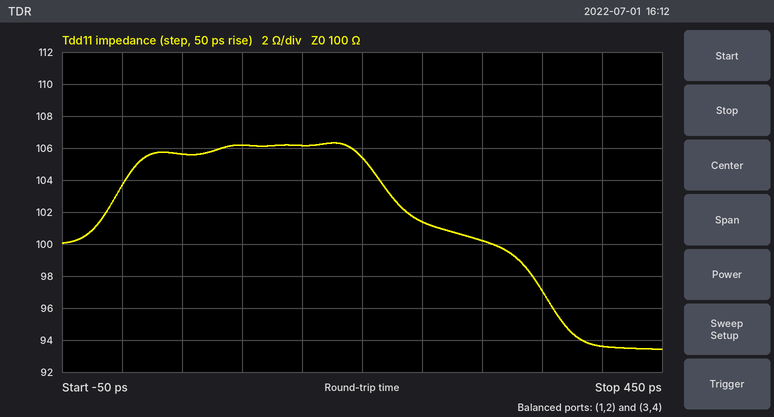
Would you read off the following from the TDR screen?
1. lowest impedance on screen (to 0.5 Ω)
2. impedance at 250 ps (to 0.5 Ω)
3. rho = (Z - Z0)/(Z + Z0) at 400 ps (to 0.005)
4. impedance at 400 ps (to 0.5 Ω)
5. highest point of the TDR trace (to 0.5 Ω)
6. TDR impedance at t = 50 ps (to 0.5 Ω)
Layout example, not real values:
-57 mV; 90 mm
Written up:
93.5 Ω; 101.5 Ω; -0.035; 93.5 Ω; 106.5 Ω; 105.5 Ω
